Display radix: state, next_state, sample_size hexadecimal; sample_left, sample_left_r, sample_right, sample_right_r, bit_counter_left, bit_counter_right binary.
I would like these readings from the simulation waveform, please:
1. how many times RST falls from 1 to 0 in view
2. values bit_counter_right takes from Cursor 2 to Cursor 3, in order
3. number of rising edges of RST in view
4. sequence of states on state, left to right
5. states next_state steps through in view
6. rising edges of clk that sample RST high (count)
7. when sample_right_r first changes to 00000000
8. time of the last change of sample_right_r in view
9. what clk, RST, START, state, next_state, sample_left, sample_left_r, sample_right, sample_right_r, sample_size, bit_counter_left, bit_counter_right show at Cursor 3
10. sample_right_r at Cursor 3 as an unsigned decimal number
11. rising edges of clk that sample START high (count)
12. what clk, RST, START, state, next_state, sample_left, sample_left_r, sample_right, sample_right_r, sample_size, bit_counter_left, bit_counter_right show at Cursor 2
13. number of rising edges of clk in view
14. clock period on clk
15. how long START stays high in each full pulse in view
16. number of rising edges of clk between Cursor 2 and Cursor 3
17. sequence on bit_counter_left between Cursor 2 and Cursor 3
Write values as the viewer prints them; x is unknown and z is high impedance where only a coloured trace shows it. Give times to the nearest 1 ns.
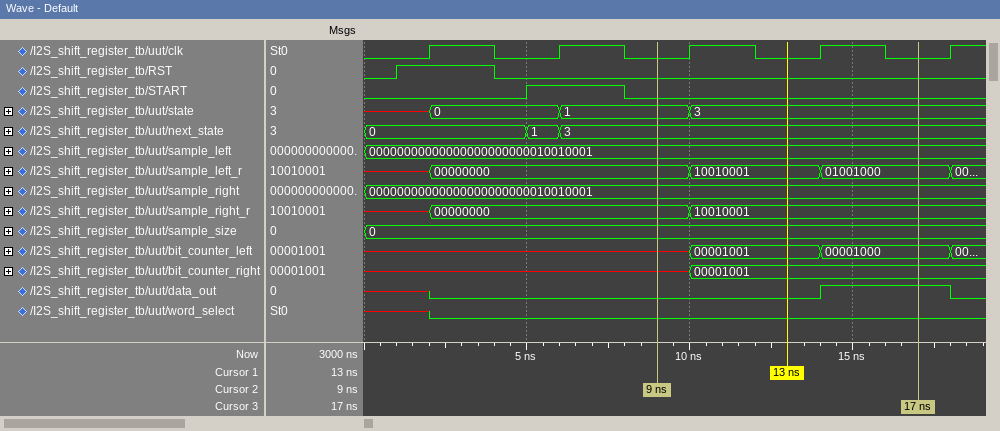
1
x, 00001001
1
x, 0, 1, 3
0, 1, 3
1
2 ns
10 ns
clk=0, RST=0, START=0, state=3, next_state=3, sample_left=00000000000000000000000010010001, sample_left_r=01001000, sample_right=00000000000000000000000010010001, sample_right_r=10010001, sample_size=0, bit_counter_left=00001000, bit_counter_right=00001001
145
1
clk=0, RST=0, START=0, state=1, next_state=3, sample_left=00000000000000000000000010010001, sample_left_r=00000000, sample_right=00000000000000000000000010010001, sample_right_r=00000000, sample_size=0, bit_counter_left=x, bit_counter_right=x
5
4 ns
3 ns
2
x, 00001001, 00001000
